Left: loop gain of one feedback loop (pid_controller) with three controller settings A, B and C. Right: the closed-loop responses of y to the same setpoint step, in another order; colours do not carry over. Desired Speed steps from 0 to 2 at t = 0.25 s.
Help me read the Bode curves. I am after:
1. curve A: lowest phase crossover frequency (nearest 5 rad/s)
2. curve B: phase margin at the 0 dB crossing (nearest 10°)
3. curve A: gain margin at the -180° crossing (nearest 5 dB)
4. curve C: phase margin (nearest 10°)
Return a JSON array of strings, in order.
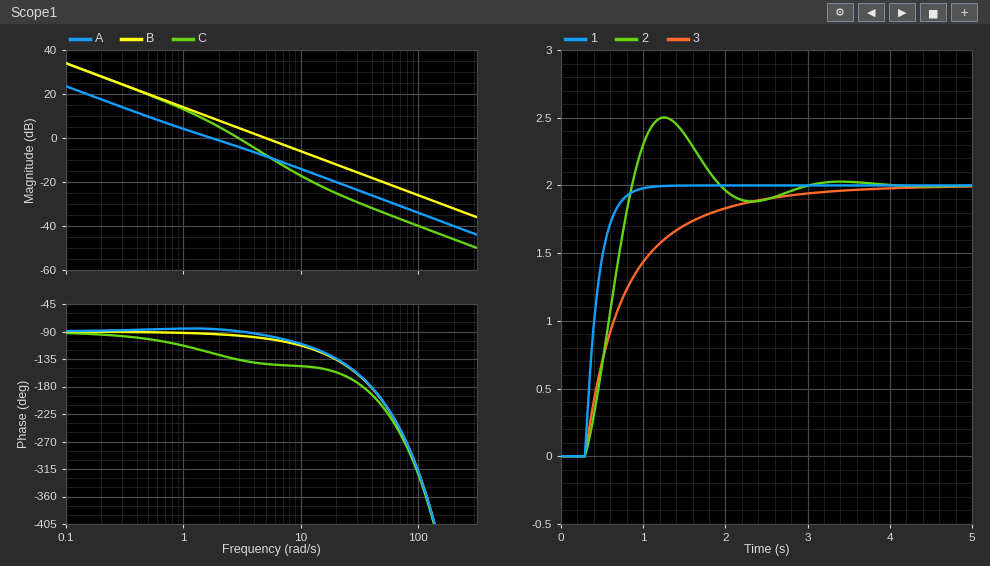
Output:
["40 rad/s", "80°", "25 dB", "40°"]
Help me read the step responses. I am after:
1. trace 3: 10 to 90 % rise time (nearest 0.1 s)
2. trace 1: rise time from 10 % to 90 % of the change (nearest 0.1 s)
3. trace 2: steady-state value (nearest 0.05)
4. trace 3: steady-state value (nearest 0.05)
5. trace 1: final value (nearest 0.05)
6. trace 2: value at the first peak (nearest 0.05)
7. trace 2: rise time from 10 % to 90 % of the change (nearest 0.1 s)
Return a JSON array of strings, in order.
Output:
["1.5 s", "0.3 s", "2.00", "2.00", "2.00", "2.50", "0.4 s"]
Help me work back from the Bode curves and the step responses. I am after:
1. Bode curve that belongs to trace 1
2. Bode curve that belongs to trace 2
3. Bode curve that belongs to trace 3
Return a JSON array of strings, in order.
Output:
["B", "C", "A"]
